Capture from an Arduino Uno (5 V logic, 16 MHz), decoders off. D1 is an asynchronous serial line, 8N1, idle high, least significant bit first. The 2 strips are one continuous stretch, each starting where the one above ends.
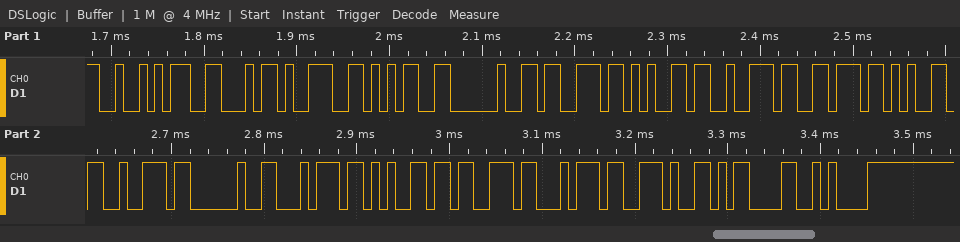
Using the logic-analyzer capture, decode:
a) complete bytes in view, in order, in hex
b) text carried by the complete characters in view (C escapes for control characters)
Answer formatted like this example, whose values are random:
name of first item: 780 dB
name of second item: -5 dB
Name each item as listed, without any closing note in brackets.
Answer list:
complete bytes in view, in order, in hex: 0x52 0x46 0x39 0x35 0x20 0x73 0x65 0x72 0x76 0x65 0x72 0x20 0x74 0x65 0x73 0x74 0x2E 0x0D 0x0A
text carried by the complete characters in view: "RF95 server test.\r\n"
